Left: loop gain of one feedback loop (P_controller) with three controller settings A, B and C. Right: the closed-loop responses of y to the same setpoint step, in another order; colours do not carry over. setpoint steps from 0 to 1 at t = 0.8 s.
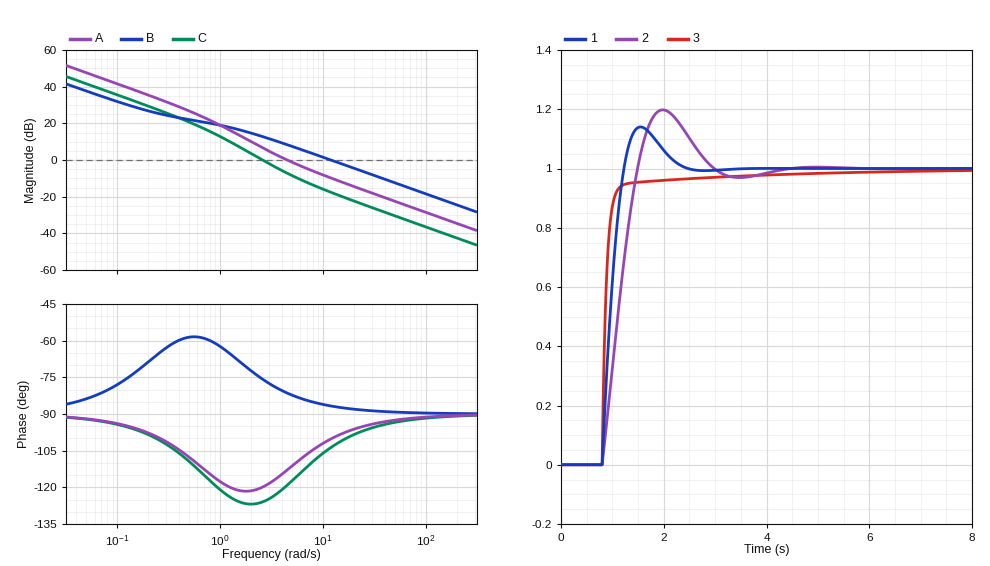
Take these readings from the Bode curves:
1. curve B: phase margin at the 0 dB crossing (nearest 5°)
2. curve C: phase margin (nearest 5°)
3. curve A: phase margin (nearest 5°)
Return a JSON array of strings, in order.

["95°", "55°", "65°"]
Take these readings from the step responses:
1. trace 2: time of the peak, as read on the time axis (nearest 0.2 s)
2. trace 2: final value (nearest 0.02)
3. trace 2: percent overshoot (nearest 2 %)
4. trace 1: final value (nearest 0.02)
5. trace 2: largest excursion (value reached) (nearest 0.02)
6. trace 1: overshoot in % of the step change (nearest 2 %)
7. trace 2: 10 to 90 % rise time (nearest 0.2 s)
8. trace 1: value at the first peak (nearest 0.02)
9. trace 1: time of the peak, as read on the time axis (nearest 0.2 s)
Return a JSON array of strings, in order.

["2.0 s", "1.00", "20 %", "1.00", "1.20", "14 %", "0.6 s", "1.14", "1.6 s"]
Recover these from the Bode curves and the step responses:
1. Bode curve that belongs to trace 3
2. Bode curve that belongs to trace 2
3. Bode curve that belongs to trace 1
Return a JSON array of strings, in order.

["B", "C", "A"]
